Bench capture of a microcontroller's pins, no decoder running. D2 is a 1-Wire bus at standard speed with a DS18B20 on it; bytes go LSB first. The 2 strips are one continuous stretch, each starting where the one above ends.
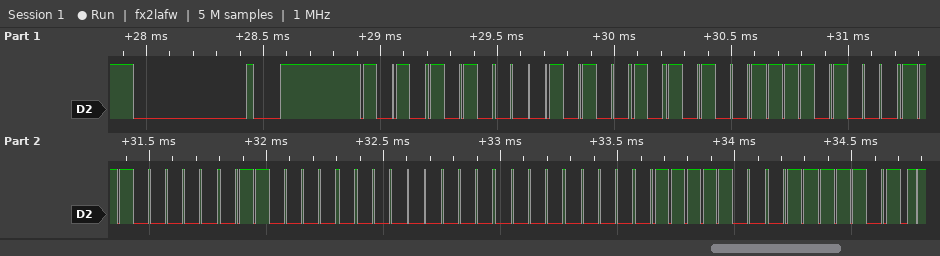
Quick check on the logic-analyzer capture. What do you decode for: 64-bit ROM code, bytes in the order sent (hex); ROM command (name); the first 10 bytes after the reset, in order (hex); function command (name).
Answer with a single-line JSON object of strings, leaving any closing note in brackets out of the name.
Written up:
{"64-bit ROM code, bytes in the order sent": "28 95 17 07 06 00 00 3E", "ROM command": "Match ROM", "the first 10 bytes after the reset, in order": "55 28 95 17 07 06 00 00 3E BE", "function command": "Read Scratchpad"}
